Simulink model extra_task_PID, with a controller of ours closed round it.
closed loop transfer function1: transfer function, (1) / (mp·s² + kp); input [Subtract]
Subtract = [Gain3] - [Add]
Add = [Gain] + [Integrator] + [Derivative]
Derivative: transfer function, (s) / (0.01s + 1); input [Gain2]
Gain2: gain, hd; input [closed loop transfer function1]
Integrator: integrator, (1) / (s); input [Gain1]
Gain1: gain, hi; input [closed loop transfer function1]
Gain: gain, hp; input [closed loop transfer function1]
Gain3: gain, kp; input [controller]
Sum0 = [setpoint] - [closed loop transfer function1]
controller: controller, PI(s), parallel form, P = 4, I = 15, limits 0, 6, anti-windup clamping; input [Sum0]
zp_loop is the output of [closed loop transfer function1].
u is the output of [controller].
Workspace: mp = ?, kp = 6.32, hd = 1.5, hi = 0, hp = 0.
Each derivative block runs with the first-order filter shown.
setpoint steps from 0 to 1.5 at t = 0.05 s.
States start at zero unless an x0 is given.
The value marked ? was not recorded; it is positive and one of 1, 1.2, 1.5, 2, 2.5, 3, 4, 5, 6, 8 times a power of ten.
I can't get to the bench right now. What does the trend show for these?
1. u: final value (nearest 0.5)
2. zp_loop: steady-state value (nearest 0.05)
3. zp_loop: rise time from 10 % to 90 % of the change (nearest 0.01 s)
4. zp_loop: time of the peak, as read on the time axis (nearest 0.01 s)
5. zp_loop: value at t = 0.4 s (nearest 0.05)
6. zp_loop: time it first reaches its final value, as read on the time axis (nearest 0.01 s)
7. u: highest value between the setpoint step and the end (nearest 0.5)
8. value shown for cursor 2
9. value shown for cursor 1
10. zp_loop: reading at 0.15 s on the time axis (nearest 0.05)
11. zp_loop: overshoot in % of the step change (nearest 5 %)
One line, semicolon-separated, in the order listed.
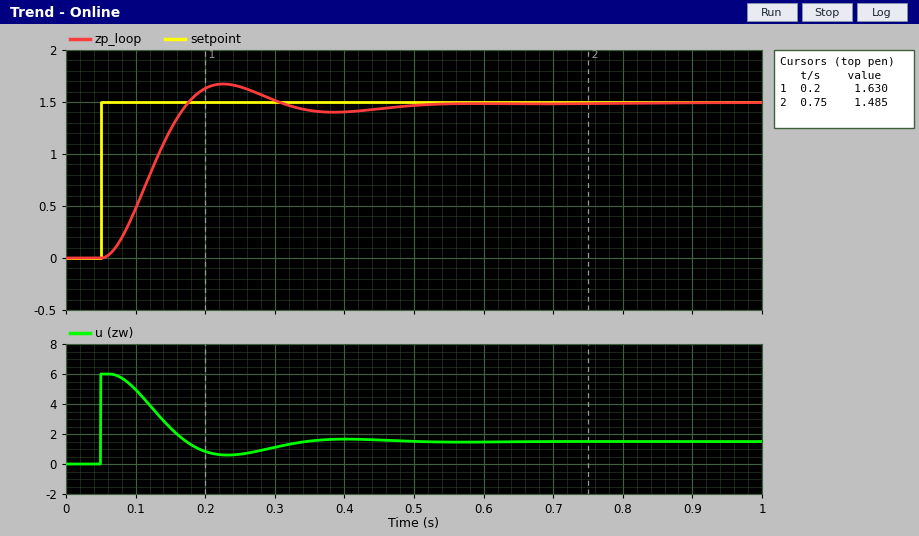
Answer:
1.5; 1.50; 0.08 s; 0.23 s; 1.40; 0.18 s; 6.0; 1.485; 1.630; 1.25; 10 %
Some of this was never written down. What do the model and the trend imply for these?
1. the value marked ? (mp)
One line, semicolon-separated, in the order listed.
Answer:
0.08
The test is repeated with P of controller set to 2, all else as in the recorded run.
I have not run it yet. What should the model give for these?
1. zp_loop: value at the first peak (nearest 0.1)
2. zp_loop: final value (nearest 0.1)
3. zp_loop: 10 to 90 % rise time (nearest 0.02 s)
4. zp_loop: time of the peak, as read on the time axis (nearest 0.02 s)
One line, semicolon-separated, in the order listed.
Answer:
1.8; 1.5; 0.12 s; 0.32 s
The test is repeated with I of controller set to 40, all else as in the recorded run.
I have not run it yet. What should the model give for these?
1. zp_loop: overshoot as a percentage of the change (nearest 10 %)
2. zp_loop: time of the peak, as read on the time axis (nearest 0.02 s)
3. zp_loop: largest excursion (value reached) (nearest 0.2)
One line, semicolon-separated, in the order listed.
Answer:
30 %; 0.22 s; 2.0
